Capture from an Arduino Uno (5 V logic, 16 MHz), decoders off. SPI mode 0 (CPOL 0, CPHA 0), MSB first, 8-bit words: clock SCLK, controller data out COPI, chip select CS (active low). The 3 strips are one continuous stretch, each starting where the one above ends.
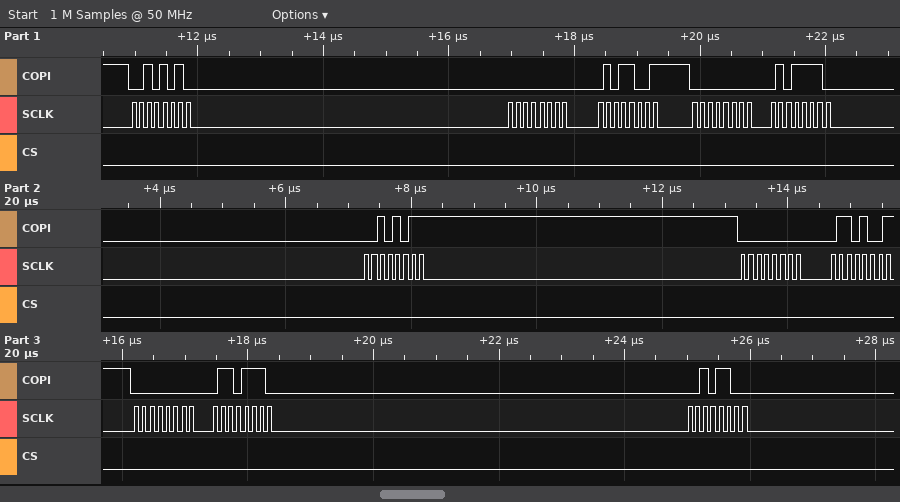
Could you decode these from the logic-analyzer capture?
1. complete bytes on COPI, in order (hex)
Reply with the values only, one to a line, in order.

2A 00 59 00 5E 2B 00 69 00 6E 2C
